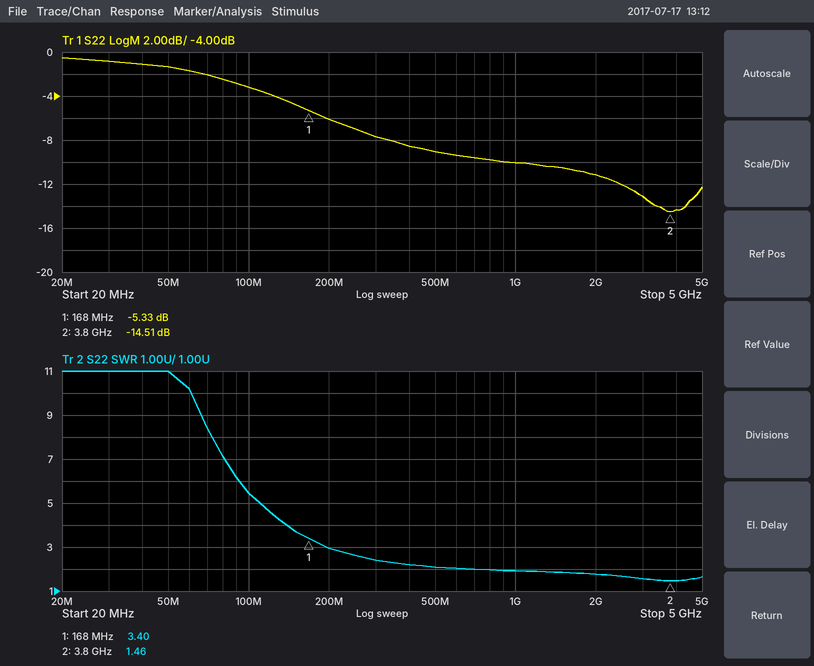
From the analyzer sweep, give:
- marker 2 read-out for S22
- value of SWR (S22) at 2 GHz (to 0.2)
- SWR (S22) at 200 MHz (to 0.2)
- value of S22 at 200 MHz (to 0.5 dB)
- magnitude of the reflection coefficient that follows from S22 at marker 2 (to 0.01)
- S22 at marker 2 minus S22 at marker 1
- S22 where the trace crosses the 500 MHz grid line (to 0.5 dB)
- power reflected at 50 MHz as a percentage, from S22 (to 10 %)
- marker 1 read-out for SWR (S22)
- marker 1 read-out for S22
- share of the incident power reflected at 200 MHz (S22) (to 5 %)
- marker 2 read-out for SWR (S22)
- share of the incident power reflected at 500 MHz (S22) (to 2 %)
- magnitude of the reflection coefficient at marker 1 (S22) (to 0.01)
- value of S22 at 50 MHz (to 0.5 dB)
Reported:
-14.51 dB
1.8
3.0
-6.0 dB
0.19
-9.18 dB
-9.0 dB
70 %
3.40
-5.33 dB
25 %
1.46
12 %
0.54
-1.5 dB
